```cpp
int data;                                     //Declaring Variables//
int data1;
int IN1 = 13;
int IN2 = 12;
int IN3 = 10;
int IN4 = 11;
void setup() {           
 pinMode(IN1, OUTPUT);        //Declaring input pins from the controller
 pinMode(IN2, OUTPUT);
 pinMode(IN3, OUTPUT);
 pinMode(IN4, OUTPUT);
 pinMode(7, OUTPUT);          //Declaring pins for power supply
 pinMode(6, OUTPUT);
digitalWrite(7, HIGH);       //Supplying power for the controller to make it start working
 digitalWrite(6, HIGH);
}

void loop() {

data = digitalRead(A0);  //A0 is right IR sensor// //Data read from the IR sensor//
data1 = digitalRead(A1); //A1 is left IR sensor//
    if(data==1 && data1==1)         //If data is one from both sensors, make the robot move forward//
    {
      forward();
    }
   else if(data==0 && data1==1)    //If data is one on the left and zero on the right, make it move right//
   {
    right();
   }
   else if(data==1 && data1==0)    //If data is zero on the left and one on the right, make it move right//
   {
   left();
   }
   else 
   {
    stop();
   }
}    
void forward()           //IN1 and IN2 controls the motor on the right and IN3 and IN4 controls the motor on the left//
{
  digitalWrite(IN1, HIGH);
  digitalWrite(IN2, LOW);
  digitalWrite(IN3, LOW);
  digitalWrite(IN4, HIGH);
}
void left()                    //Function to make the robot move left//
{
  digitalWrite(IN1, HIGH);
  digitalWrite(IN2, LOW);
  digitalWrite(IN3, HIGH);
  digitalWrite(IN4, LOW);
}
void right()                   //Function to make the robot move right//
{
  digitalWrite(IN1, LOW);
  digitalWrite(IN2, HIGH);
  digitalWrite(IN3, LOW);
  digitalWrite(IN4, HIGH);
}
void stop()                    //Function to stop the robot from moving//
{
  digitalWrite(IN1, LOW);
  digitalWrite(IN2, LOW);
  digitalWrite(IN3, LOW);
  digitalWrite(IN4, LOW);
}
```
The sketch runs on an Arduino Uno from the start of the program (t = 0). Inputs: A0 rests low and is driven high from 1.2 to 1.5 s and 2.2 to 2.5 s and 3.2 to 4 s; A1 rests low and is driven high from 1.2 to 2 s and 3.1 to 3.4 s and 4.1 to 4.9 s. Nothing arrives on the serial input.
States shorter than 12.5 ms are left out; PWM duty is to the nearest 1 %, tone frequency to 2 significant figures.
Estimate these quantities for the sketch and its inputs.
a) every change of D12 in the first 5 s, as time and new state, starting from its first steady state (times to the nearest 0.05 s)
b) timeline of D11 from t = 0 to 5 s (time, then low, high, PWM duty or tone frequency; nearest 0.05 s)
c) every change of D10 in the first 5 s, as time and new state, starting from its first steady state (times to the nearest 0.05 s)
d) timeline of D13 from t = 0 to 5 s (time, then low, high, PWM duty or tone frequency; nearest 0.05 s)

0 s low; 1.5 s high; 2 s low; 3.1 s high; 3.2 s low; 4.1 s high; 4.9 s low
0 s low; 1.2 s high; 2 s low; 3.1 s high; 3.4 s low; 4.1 s high; 4.9 s low
0 s low; 2.2 s high; 2.5 s low; 3.4 s high; 4 s low
0 s low; 1.2 s high; 1.5 s low; 2.2 s high; 2.5 s low; 3.2 s high; 4 s low
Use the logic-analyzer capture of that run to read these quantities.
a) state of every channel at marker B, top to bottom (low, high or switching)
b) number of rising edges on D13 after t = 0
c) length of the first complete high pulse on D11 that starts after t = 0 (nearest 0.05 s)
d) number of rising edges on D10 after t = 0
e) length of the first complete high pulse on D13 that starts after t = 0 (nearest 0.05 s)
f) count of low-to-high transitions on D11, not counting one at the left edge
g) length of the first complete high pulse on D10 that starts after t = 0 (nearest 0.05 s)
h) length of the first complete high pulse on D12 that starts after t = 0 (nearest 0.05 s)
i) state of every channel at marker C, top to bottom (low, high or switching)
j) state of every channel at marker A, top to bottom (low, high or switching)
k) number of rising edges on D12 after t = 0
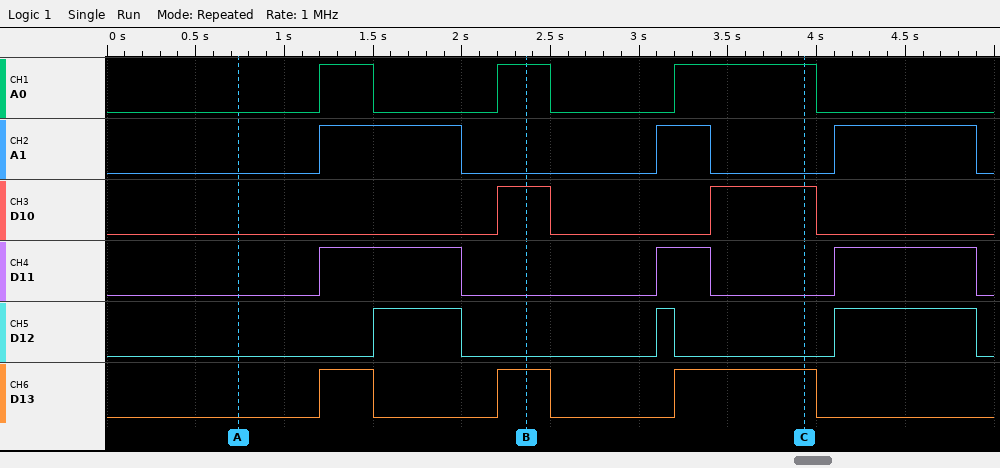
A0 high, A1 low, D10 high, D11 low, D12 low, D13 high
3
0.80 s
2
0.30 s
3
0.30 s
0.50 s
A0 high, A1 low, D10 high, D11 low, D12 low, D13 high
A0 low, A1 low, D10 low, D11 low, D12 low, D13 low
3
